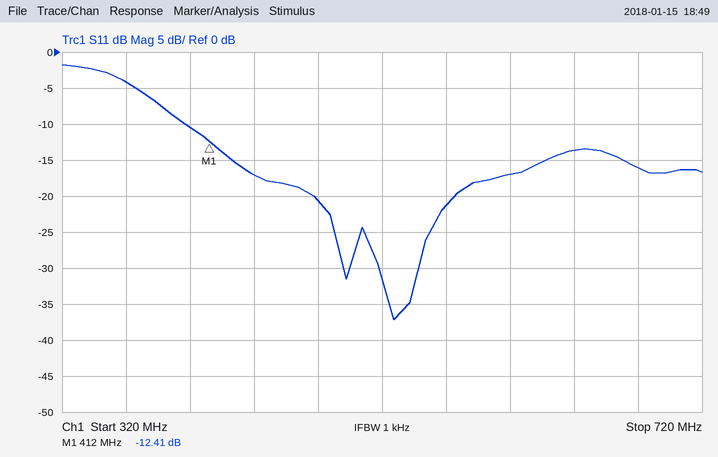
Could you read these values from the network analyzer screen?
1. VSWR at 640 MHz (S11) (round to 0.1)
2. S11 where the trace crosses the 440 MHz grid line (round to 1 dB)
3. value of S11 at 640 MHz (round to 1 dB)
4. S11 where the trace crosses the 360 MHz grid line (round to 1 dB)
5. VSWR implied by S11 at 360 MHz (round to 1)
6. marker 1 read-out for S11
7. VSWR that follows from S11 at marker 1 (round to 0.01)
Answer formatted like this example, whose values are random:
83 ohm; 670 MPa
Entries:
1.5; -17 dB; -14 dB; -4 dB; 4; -12.41 dB; 1.63
